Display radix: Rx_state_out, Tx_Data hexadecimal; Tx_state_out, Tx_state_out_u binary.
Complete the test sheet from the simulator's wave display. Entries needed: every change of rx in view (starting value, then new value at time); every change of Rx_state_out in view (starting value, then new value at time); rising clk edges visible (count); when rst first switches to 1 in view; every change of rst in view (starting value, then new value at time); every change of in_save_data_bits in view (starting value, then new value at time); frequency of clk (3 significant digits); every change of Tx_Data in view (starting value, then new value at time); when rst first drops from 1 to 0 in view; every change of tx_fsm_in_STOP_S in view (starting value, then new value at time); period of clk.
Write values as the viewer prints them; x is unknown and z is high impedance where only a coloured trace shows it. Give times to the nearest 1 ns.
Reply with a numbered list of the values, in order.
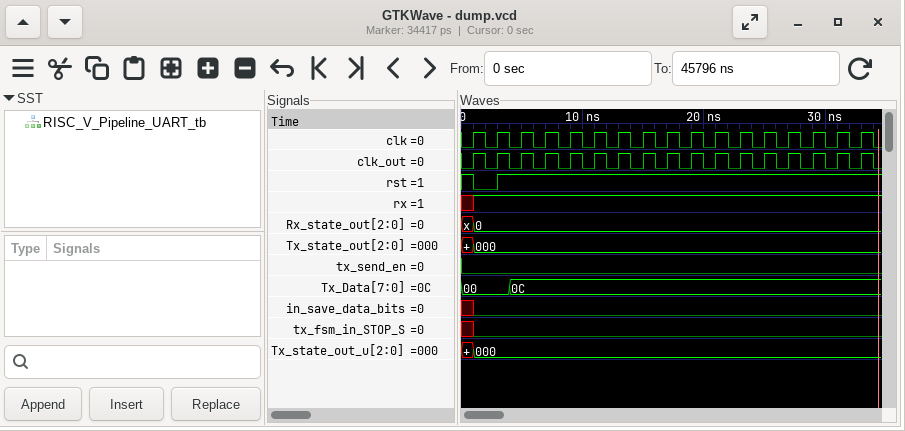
1. x, 1 at 1 ns
2. x, 0 at 1 ns
3. 17
4. 3 ns
5. 1, 0 at 1 ns, 1 at 3 ns
6. x, 0 at 1 ns
7. 500 MHz
8. 00, 0C at 4 ns
9. 1 ns
10. x, 0 at 1 ns
11. 2 ns
